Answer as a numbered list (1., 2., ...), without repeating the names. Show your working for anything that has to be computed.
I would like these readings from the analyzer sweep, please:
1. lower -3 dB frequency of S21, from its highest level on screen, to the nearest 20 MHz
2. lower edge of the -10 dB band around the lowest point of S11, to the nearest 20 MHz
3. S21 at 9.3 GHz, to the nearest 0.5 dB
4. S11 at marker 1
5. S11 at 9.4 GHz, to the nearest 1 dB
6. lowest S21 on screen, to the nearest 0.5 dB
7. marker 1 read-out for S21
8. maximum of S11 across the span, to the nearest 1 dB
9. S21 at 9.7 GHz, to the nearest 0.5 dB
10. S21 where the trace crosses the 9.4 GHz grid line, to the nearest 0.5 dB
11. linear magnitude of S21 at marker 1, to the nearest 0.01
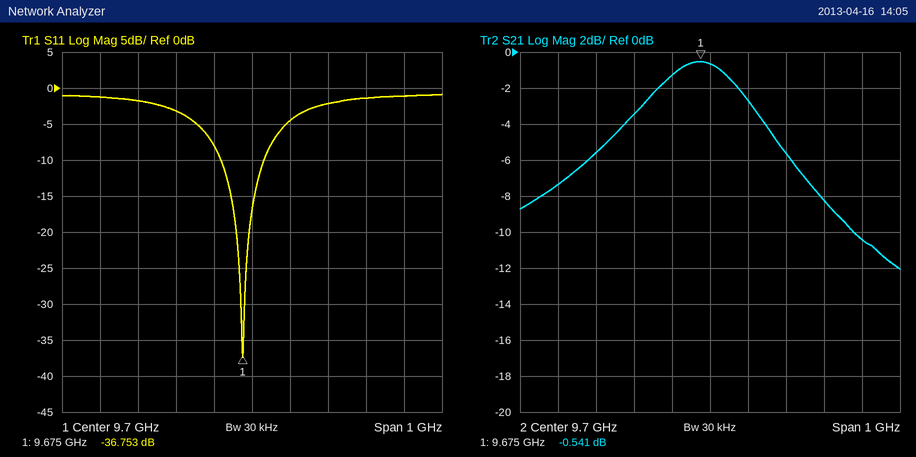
1. 9.50 GHz
2. 9.62 GHz
3. -7.5 dB
4. -36.753 dB
5. -2 dB
6. -12.0 dB
7. -0.541 dB
8. -1 dB
9. -0.5 dB
10. -5.5 dB
11. 10^(-0.541/20) ≈ 0.94
